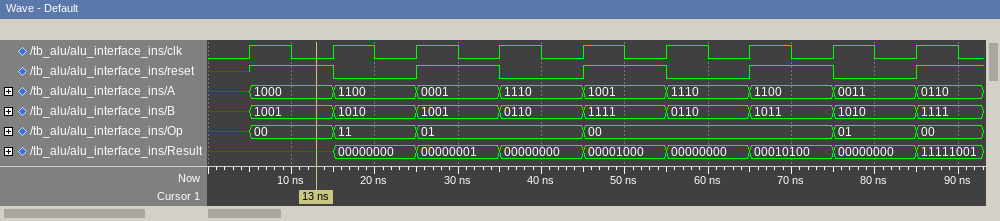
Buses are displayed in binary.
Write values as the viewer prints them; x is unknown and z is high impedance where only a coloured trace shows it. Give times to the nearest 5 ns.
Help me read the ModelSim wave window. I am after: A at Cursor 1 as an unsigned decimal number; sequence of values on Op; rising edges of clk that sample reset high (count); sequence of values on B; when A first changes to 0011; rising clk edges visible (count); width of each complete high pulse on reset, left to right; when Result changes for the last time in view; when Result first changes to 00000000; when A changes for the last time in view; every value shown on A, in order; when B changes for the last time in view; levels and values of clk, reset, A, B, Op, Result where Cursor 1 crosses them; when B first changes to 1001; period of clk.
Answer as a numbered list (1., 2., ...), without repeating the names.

1. 8
2. x, 00, 11, 01, 00, 01, 00
3. 4
4. x, 1001, 1010, 1001, 0110, 1111, 0110, 1011, 1010, 1111
5. 75 ns
6. 9
7. 10 ns, 10 ns, 10 ns
8. 85 ns
9. 15 ns
10. 85 ns
11. x, 1000, 1100, 0001, 1110, 1001, 1110, 1100, 0011, 0110
12. 85 ns
13. clk=0, reset=1, A=1000, B=1001, Op=00, Result=x
14. 5 ns
15. 10 ns
